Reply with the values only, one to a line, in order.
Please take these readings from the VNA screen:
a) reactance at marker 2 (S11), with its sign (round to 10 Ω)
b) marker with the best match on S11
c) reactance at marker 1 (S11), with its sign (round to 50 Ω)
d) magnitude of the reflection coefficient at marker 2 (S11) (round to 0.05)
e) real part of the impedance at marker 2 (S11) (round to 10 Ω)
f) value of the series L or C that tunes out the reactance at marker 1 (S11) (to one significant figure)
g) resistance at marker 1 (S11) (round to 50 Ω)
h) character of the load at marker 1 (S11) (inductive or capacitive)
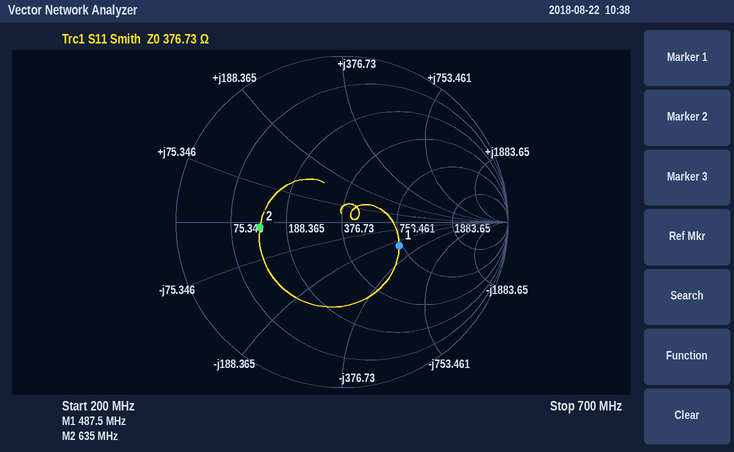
-10 Ω
marker 1
-250 Ω
0.50
130 Ω
80 nH
700 Ω
capacitive
